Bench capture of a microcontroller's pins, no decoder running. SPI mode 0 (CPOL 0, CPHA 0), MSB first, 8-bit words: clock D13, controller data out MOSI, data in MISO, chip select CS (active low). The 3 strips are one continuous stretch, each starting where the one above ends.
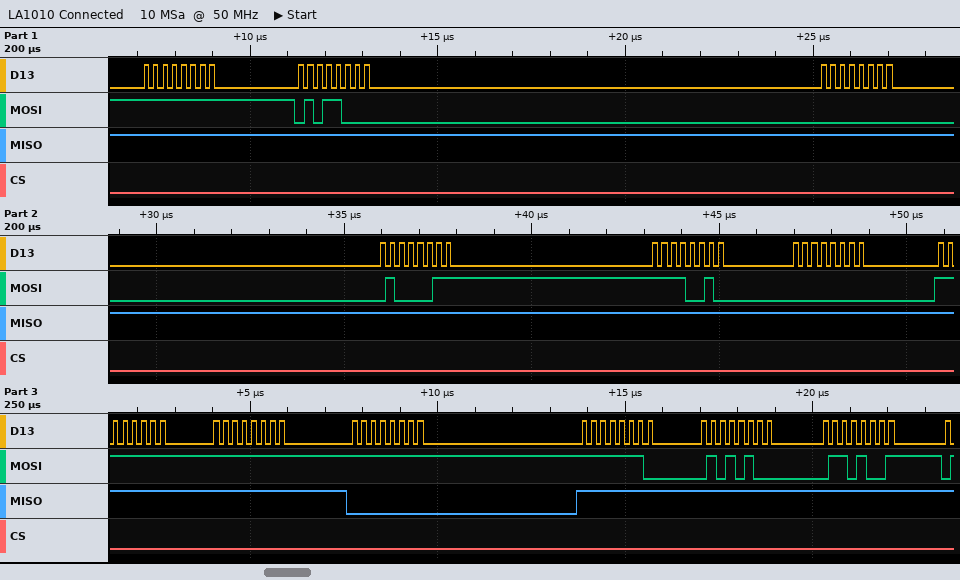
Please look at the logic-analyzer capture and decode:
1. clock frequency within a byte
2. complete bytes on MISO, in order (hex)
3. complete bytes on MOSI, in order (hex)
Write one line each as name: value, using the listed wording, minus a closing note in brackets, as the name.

clock frequency within a byte: 4 MHz
complete bytes on MISO, in order: 0xFF 0xFF 0xFF 0xFF 0xFF 0xFF 0xFF 0xFF 0x00 0xFF 0xFF 0xFF
complete bytes on MOSI, in order: 0xFF 0x58 0x00 0x43 0xF2 0x00 0xFF 0xFF 0xFF 0xFE 0x54 0x69
